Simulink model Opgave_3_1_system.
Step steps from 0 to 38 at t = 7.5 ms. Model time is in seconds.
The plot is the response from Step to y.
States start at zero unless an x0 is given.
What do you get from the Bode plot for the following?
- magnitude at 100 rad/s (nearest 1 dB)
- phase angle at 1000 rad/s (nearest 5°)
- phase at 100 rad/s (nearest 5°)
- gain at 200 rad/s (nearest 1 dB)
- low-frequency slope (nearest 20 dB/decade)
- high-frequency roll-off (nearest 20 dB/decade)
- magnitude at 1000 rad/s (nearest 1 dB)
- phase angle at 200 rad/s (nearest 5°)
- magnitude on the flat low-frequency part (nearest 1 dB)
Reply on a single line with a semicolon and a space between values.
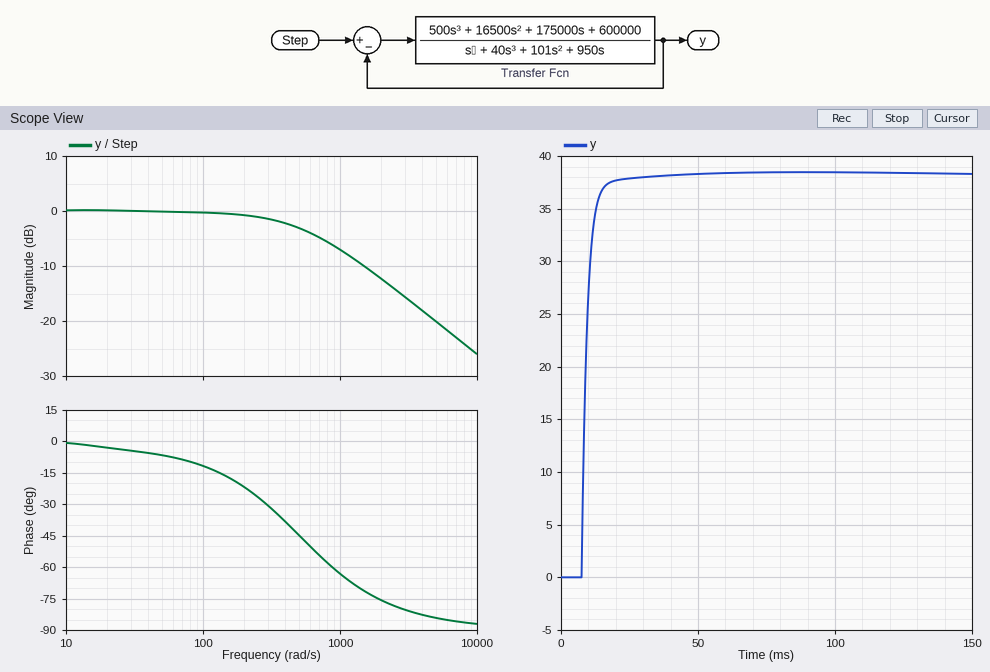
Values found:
0 dB; -65°; -10°; -1 dB; 0 dB/decade; -20 dB/decade; -7 dB; -20°; 0 dB
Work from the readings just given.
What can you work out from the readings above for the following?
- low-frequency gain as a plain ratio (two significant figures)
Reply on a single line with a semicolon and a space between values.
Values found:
1.0
